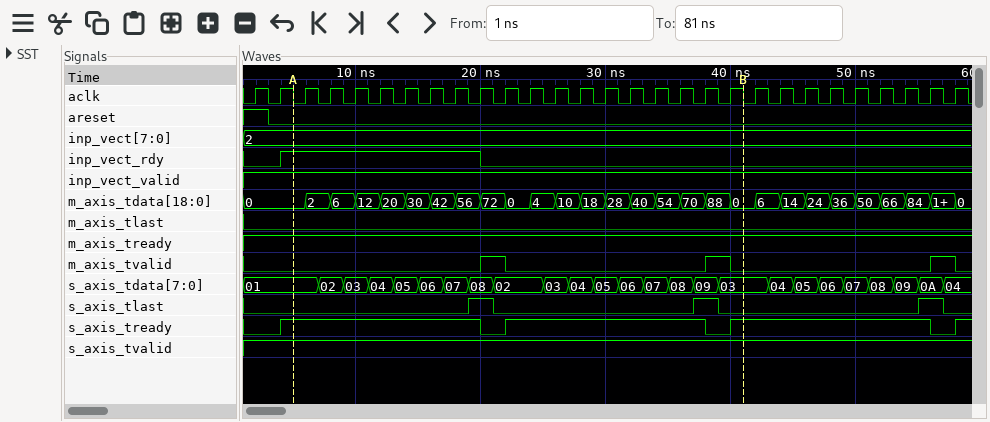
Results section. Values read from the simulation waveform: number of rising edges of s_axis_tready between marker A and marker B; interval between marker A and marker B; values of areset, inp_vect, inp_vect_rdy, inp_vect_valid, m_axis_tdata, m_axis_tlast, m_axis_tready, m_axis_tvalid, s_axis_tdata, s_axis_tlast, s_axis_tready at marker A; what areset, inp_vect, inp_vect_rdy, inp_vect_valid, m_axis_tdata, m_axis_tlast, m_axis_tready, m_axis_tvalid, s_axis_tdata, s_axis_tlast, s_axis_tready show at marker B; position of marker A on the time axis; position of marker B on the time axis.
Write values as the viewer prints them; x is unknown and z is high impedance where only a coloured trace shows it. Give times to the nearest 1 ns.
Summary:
2
36 ns
areset=0, inp_vect=2, inp_vect_rdy=1, inp_vect_valid=1, m_axis_tdata=0, m_axis_tlast=0, m_axis_tready=1, m_axis_tvalid=0, s_axis_tdata=01, s_axis_tlast=0, s_axis_tready=1
areset=0, inp_vect=2, inp_vect_rdy=0, inp_vect_valid=1, m_axis_tdata=0, m_axis_tlast=0, m_axis_tready=1, m_axis_tvalid=0, s_axis_tdata=03, s_axis_tlast=0, s_axis_tready=1
5 ns
41 ns
